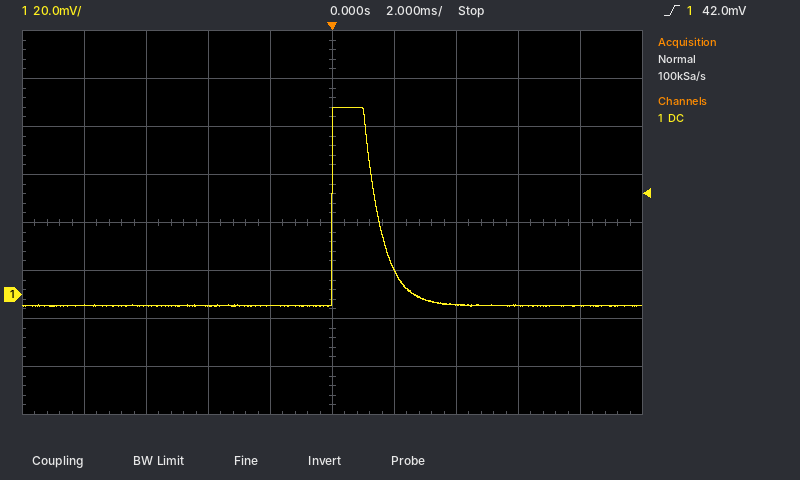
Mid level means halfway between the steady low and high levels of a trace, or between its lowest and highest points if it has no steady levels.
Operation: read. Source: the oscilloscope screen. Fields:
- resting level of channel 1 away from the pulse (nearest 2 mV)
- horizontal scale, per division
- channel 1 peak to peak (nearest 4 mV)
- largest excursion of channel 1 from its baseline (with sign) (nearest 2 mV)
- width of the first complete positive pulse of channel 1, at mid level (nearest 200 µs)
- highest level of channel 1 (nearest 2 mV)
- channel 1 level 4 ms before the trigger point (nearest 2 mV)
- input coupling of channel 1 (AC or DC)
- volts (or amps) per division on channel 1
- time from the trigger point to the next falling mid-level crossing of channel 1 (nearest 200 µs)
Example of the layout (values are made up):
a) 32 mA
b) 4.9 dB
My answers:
a) -4 mV
b) 2 ms
c) 84 mV
d) +82 mV
e) 1.4 ms
f) 78 mV
g) -4 mV
h) DC
i) 20 mV
j) 1.4 ms
